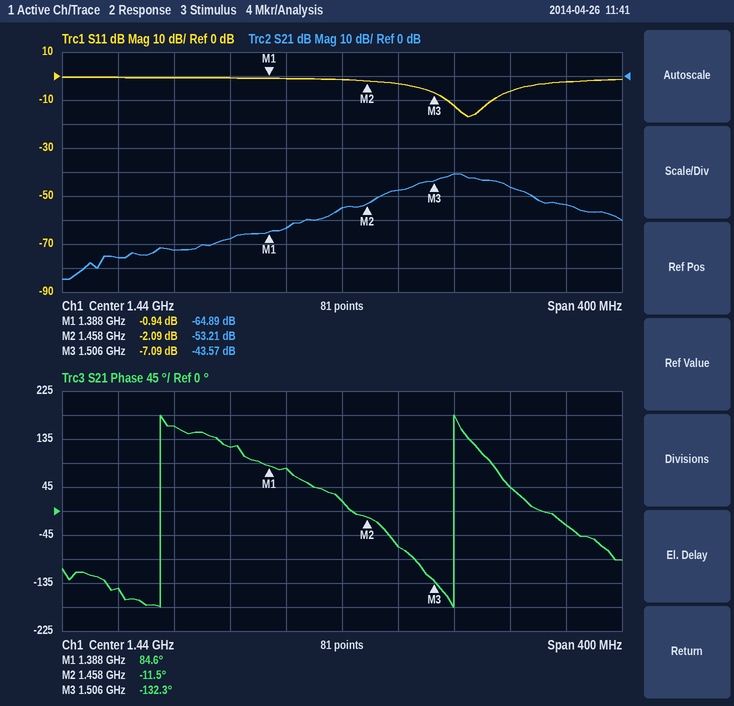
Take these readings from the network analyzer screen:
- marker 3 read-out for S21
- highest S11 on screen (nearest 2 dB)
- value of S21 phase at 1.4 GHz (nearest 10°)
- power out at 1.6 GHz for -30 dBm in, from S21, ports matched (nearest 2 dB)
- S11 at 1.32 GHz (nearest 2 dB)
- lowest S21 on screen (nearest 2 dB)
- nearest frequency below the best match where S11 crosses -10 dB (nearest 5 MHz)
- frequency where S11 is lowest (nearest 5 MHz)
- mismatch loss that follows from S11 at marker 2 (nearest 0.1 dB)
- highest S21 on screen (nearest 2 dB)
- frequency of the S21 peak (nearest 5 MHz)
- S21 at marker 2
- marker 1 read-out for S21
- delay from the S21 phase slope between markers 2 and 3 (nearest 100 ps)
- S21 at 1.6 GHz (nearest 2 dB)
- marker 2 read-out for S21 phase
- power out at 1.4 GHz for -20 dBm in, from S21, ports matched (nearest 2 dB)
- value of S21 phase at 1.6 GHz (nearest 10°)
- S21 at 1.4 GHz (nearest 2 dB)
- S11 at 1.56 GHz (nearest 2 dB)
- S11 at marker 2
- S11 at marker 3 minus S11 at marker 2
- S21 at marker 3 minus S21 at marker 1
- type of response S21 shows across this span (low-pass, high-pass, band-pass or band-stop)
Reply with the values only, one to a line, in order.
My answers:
-43.57 dB
0 dB
80°
-84 dBm
0 dB
-84 dB
1.515 GHz
1.530 GHz
4.2 dB
-40 dB
1.520 GHz
-53.21 dB
-64.89 dB
7.0 ns
-54 dB
-11.5°
-84 dBm
-30°
-64 dB
-6 dB
-2.09 dB
-5.00 dB
21.32 dB
band-pass
